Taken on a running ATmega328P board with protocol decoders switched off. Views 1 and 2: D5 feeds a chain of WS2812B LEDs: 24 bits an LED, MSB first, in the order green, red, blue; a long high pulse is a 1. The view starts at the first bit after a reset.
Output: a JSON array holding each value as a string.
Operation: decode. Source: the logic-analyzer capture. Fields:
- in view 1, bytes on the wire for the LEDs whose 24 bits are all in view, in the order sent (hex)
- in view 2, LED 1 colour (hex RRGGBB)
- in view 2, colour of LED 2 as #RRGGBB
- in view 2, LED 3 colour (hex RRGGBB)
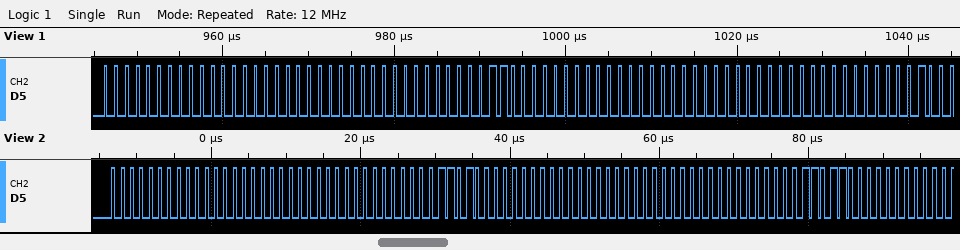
["00 00 00 00 0C 00 00 00 00", "#000000", "#1A0000", "#000000"]
